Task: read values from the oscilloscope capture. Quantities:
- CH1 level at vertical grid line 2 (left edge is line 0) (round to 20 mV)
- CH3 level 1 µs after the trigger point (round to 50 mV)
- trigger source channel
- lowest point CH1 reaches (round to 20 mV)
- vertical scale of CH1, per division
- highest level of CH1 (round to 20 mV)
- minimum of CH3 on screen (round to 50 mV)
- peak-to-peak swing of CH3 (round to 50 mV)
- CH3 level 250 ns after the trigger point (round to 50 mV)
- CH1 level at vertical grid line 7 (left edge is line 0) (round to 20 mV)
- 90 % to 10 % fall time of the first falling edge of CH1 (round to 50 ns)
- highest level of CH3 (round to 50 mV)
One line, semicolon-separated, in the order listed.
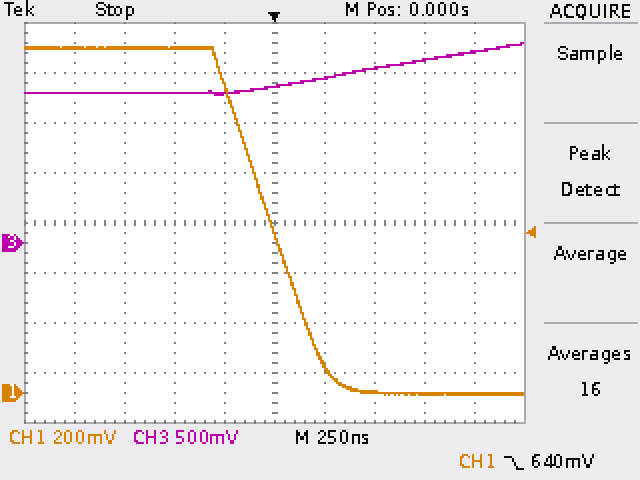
1.38 V; 1.90 V; CH1; 0 mV; 200 mV; 1.38 V; 1.50 V; 500 mV; 1.65 V; 0 mV; 500 ns; 2.00 V
